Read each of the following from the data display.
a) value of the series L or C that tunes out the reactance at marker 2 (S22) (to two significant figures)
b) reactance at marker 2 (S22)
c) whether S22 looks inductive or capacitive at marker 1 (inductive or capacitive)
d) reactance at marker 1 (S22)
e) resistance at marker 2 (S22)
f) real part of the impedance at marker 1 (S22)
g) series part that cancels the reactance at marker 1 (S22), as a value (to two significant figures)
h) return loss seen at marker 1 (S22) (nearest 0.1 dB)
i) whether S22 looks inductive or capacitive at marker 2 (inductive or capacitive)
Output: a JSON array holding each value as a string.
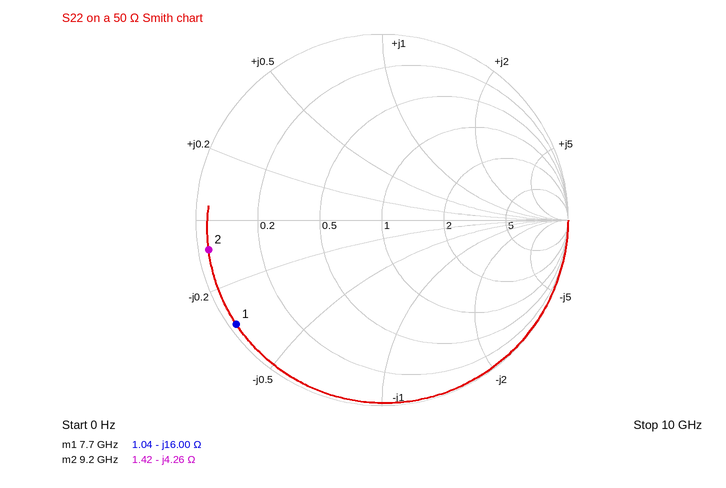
["74 pH", "-4.26 Ω", "capacitive", "-16.00 Ω", "1.42 Ω", "1.04 Ω", "330 pH", "0.3 dB", "capacitive"]
